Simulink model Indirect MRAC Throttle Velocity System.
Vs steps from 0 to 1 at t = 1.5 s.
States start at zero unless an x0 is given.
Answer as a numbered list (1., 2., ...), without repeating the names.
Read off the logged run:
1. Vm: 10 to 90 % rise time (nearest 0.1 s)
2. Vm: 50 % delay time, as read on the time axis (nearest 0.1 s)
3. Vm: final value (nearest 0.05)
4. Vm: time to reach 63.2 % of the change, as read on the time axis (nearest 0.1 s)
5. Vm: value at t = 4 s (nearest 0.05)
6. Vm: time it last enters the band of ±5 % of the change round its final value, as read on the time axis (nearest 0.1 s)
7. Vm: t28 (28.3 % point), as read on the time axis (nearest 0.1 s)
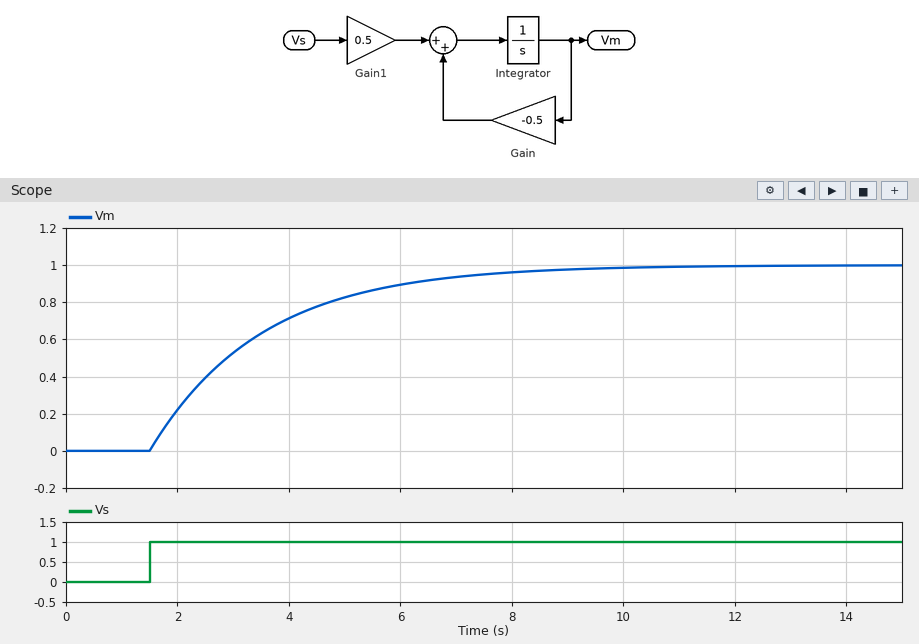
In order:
1. 4.4 s
2. 2.9 s
3. 1.00
4. 3.5 s
5. 0.70
6. 7.5 s
7. 2.2 s
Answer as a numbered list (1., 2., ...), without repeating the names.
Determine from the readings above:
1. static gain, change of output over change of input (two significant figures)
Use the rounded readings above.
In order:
1. 1.0
